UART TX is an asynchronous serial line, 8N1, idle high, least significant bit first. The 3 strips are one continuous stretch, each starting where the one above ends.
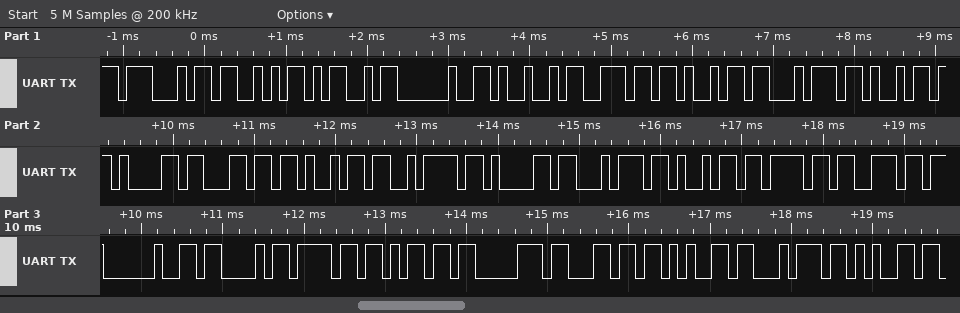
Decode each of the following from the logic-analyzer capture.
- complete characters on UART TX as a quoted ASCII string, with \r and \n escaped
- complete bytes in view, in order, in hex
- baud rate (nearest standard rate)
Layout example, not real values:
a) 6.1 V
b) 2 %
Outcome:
a) "GSM Initialization Complete"
b) 47 53 4D 20 49 6E 69 74 69 61 6C 69 7A 61 74 69 6F 6E 20 43 6F 6D 70 6C 65 74 65
c) 9600 baud
